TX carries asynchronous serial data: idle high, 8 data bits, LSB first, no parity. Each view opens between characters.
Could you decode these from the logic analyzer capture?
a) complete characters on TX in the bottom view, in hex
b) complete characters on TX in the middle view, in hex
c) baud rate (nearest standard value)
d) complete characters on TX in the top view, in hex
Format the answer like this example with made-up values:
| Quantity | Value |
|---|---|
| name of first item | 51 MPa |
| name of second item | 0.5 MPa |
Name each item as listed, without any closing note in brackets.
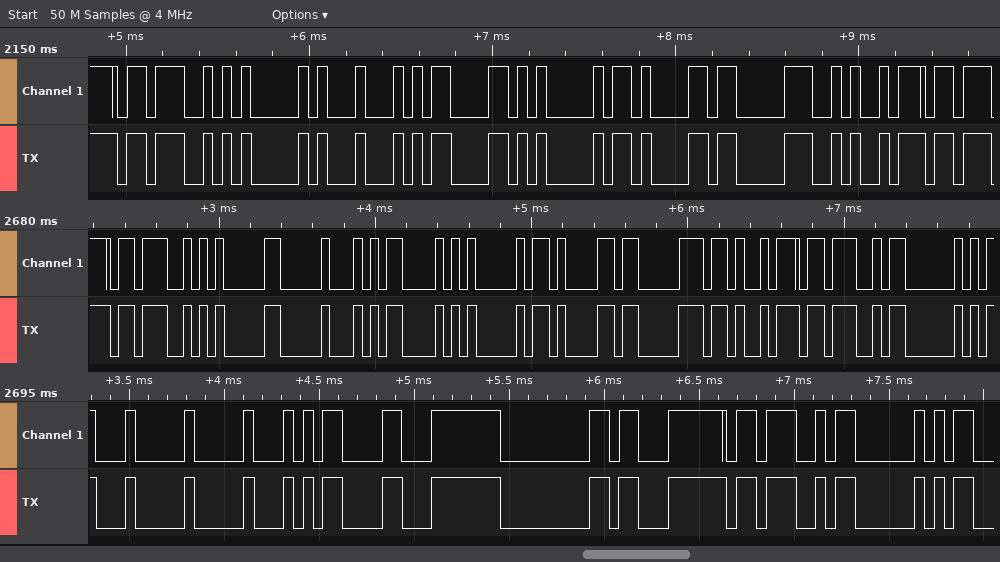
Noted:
| Quantity | Value |
|---|---|
| complete characters on TX in the bottom view, in hex | 04, 10, 0D, FC, 00, E3, 3B, 03 |
| complete characters on TX in the middle view, in hex | 3B, 05, 10, 0D, 05, 0B, 83, 4B, 3B, 03 |
| baud rate | 19200 baud |
| complete characters on TX in the top view, in hex | 3B, 05, 11, 0D, 05, 0B, 83, 4A |
